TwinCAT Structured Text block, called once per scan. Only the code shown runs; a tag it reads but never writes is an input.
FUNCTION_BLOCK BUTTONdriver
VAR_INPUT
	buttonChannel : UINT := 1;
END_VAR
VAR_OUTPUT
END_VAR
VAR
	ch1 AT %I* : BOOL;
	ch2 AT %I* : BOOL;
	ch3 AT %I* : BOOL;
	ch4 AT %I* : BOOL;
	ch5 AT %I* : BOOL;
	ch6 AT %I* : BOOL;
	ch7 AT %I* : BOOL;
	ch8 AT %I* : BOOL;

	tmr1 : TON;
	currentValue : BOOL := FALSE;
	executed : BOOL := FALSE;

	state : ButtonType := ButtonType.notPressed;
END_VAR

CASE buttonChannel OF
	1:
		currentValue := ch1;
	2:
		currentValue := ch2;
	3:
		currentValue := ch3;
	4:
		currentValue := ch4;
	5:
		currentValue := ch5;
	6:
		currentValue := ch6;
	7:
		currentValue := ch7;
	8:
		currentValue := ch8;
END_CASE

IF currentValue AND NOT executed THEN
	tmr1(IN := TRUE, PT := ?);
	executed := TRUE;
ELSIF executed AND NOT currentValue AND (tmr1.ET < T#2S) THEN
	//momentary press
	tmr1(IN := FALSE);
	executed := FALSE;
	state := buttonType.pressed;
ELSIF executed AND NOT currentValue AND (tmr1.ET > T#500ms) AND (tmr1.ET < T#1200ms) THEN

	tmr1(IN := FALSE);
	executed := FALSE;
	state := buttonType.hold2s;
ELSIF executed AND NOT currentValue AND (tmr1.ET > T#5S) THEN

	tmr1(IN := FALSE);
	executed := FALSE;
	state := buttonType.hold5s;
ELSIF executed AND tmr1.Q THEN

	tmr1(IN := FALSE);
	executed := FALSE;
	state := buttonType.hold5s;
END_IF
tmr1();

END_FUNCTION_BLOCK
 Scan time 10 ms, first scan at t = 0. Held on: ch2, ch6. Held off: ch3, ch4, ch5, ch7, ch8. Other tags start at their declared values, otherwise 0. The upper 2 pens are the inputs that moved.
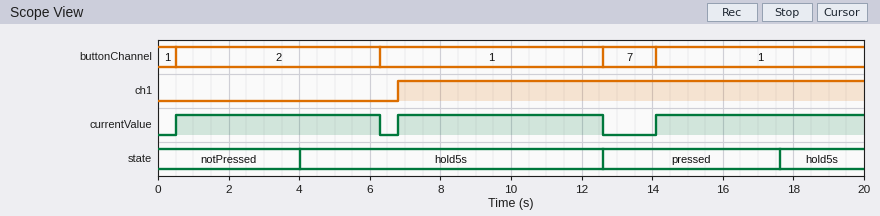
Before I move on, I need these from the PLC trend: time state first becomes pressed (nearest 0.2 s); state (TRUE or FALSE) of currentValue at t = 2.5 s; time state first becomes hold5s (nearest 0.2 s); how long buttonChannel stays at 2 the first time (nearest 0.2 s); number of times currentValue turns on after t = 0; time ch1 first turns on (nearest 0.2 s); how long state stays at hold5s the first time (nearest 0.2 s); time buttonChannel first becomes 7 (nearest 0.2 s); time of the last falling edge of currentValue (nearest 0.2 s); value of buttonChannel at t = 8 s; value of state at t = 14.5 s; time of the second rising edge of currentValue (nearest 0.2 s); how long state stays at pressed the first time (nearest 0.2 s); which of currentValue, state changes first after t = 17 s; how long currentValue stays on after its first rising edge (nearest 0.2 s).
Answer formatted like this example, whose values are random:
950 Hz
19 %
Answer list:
12.6 s
TRUE
4.0 s
5.8 s
3
6.8 s
8.6 s
12.6 s
12.6 s
1
pressed
6.8 s
5.0 s
state
5.8 s
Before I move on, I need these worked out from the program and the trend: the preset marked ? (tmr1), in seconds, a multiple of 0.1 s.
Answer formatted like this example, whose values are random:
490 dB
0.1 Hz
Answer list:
3.5 s
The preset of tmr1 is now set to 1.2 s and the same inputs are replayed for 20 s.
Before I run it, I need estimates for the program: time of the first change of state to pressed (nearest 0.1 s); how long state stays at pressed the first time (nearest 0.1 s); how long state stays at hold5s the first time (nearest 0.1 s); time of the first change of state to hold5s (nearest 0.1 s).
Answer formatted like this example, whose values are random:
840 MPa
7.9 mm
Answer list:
6.3 s
1.7 s
4.6 s
1.7 s
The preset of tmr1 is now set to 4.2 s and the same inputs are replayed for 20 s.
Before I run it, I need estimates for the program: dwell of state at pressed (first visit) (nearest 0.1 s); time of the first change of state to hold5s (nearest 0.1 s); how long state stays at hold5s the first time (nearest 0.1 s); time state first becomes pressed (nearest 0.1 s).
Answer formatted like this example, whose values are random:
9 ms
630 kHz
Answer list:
4.7 s
4.7 s
1.6 s
6.3 s
